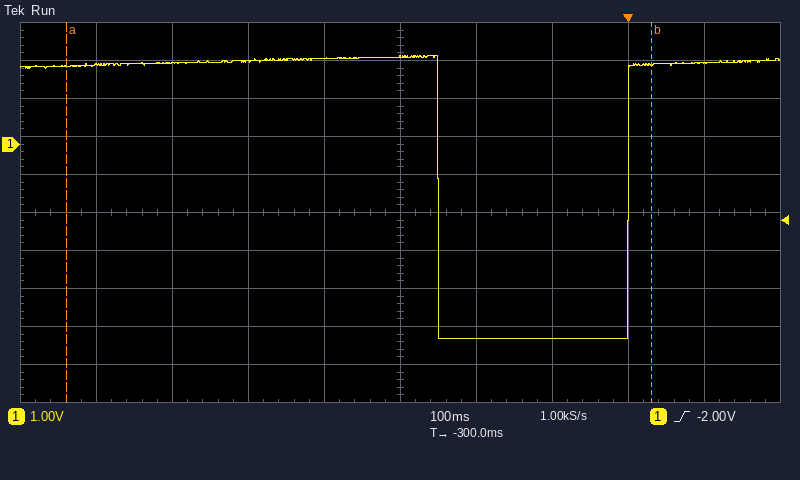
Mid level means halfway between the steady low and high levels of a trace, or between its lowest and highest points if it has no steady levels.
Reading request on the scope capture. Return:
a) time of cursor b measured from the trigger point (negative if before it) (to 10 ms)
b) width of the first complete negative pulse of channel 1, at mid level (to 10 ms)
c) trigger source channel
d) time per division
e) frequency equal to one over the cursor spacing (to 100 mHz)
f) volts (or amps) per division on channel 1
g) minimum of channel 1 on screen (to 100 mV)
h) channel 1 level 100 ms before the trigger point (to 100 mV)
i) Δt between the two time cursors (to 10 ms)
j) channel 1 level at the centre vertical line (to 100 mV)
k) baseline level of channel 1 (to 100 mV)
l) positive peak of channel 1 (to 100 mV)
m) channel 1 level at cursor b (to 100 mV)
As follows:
+30 ms
250 ms
channel 1
100 ms
1.3 Hz
1 V
-5.1 V
-5.1 V
770 ms
2.3 V
2.1 V
2.3 V
2.1 V
